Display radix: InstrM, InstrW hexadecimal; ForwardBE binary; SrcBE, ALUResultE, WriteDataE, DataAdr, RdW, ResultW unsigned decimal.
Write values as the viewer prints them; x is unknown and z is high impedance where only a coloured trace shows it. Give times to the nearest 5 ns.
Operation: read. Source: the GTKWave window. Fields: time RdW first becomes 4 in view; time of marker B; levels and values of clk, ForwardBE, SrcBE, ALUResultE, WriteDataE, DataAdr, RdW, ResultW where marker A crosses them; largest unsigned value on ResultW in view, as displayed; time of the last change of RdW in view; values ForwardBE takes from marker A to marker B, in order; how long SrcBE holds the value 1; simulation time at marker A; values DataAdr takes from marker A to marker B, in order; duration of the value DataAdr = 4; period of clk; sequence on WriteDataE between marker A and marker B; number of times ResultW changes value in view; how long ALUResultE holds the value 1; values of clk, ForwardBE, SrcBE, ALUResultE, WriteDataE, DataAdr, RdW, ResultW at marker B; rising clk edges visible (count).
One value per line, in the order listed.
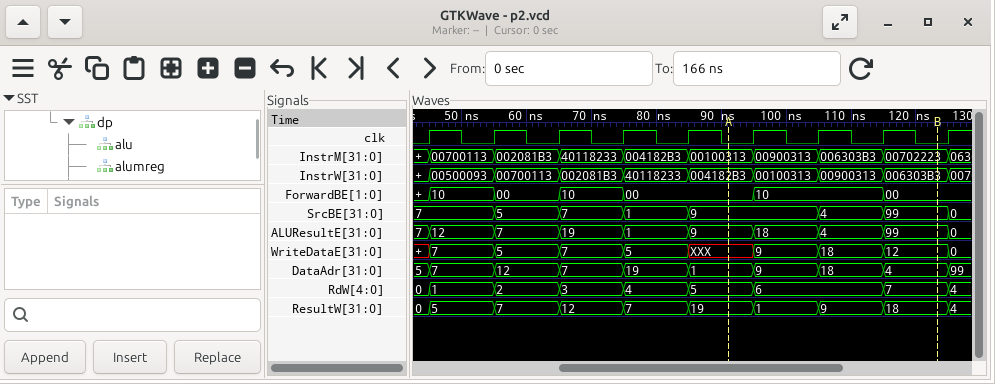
75 ns
125 ns
clk=0, ForwardBE=00, SrcBE=9, ALUResultE=9, WriteDataE=XXX, DataAdr=1, RdW=5, ResultW=19
19
125 ns
00, 10, 00
10 ns
90 ns
1, 9, 18, 4
10 ns
10 ns
XXX, 9, 18, 12
9
10 ns
clk=0, ForwardBE=00, SrcBE=99, ALUResultE=99, WriteDataE=12, DataAdr=4, RdW=7, ResultW=18
9
